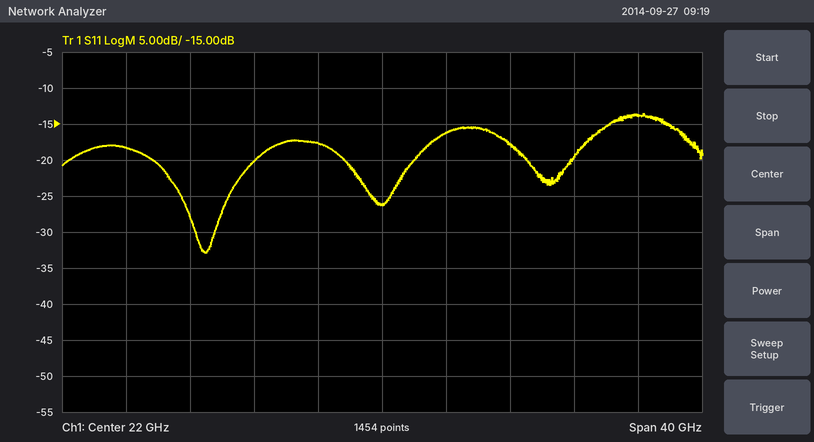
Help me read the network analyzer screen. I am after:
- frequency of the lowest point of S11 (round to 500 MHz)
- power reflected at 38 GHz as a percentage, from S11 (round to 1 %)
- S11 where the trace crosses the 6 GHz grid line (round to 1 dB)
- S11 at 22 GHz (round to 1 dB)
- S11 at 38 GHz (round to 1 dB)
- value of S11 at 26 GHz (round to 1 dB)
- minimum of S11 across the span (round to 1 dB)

11.0 GHz
4 %
-18 dB
-26 dB
-14 dB
-16 dB
-33 dB
